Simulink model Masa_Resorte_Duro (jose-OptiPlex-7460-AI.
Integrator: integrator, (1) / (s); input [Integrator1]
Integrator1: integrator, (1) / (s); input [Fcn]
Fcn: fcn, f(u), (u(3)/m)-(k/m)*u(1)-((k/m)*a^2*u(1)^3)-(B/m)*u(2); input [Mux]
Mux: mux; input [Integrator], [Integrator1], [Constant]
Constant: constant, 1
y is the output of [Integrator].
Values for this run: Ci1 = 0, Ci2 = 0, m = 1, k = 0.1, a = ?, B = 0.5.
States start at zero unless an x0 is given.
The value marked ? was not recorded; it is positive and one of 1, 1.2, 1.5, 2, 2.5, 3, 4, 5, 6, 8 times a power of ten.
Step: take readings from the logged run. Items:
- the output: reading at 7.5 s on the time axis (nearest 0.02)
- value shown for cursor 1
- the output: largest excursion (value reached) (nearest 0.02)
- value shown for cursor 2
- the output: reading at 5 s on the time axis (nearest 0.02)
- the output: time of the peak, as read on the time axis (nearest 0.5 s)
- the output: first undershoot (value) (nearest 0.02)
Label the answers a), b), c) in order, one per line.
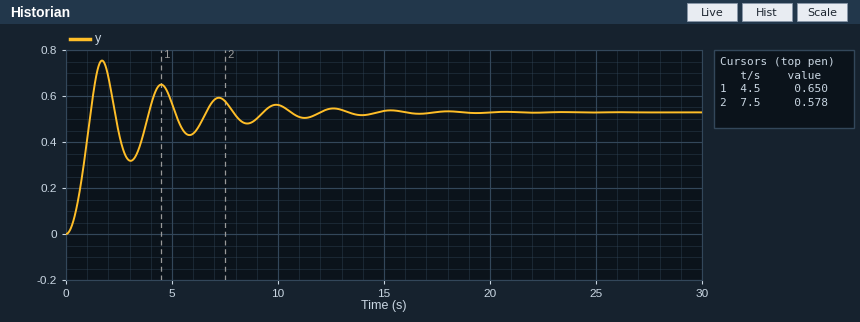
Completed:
a) 0.58
b) 0.650
c) 0.76
d) 0.578
e) 0.56
f) 1.5 s
g) 0.32
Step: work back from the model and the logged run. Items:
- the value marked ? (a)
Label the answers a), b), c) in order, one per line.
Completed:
a) 8
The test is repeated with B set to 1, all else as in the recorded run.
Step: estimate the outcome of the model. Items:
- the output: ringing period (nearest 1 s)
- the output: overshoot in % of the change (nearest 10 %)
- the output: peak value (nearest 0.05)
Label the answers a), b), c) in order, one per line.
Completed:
a) 3 s
b) 30 %
c) 0.70
